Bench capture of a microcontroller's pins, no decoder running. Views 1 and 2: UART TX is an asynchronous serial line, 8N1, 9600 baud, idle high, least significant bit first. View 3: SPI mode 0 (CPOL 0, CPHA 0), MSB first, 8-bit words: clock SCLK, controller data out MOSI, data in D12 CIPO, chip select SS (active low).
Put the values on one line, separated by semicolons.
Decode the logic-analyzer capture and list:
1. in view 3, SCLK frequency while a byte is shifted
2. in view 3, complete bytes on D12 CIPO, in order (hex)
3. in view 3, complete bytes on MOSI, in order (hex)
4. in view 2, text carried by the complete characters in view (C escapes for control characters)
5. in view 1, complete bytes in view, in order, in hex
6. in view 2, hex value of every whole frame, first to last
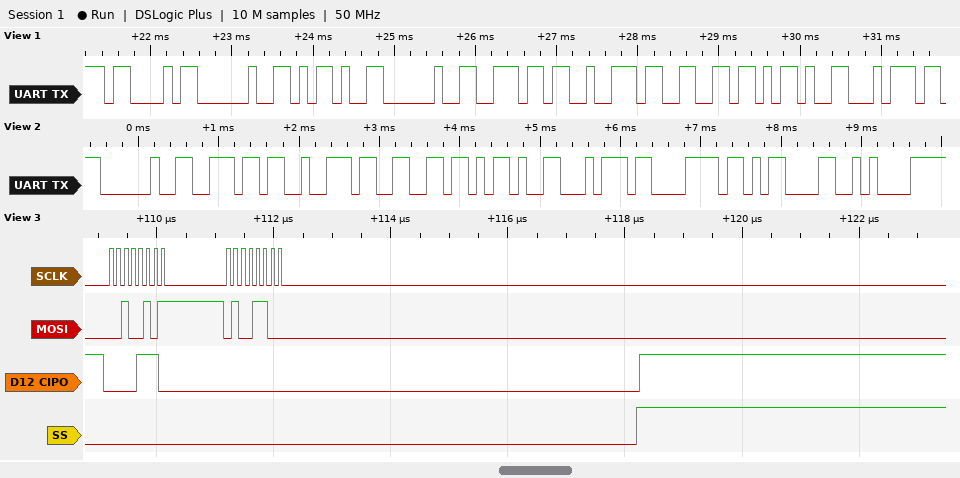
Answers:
8 MHz; 0E 00; 25 4C; " nrf-tx\r\n"; 43 20 2D 20 6E 72 66 2D 74; 0x20 0x6E 0x72 0x66 0x2D 0x74 0x78 0x0D 0x0A
